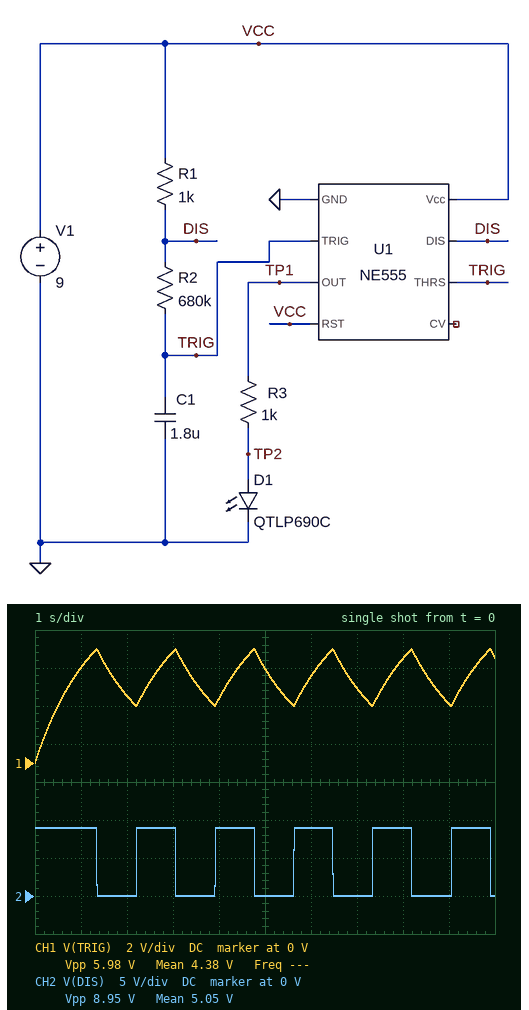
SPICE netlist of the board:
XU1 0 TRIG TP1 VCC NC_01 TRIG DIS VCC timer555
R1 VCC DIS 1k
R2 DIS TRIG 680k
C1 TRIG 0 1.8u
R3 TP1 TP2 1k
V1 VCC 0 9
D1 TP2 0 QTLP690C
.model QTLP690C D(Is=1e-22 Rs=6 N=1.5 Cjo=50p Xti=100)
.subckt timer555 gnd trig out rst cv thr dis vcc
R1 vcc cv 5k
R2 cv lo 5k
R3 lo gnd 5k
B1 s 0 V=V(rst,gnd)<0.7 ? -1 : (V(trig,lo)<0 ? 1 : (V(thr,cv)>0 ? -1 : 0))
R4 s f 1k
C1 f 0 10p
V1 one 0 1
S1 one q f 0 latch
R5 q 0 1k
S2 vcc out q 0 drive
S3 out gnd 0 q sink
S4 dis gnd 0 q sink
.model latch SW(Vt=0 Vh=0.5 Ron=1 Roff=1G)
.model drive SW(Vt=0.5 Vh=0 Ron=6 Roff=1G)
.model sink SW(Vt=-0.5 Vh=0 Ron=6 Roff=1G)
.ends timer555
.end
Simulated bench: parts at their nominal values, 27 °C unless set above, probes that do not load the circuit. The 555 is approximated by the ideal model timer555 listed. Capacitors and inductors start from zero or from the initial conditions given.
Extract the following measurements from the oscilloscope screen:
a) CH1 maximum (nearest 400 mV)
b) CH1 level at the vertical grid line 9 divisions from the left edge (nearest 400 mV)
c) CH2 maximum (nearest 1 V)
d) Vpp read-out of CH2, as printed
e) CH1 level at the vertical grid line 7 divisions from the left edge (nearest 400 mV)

6.0 V
3.2 V
9 V
8.95 V
4.0 V
